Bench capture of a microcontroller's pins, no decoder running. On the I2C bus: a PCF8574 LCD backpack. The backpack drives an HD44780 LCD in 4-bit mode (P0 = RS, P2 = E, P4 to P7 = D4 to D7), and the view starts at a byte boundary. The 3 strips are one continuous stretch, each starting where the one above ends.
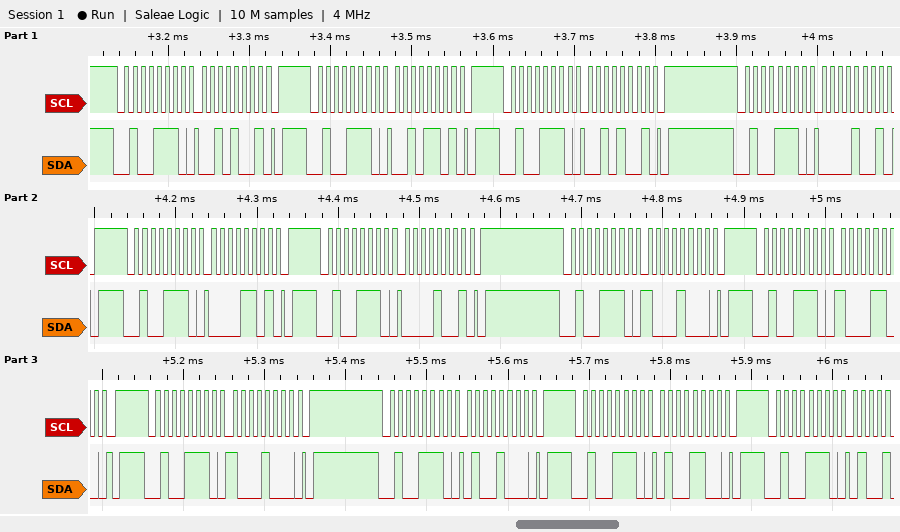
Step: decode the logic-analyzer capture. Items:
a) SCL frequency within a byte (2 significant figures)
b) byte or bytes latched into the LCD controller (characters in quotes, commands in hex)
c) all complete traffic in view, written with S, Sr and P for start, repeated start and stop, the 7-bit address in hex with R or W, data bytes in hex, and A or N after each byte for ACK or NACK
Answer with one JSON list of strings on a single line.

["100 kHz", "' '", "S 27W A 29 A P S 27W A 2D A P S 27W A 29 A P S 27W A 09 A P S 27W A 0D A P S 27W A 09 A P S 27W A 88 A P S 27W A 8C A P S 27W A 88 A P S 27W A 48 A P S 27W A 4C A P S 27W A"]
